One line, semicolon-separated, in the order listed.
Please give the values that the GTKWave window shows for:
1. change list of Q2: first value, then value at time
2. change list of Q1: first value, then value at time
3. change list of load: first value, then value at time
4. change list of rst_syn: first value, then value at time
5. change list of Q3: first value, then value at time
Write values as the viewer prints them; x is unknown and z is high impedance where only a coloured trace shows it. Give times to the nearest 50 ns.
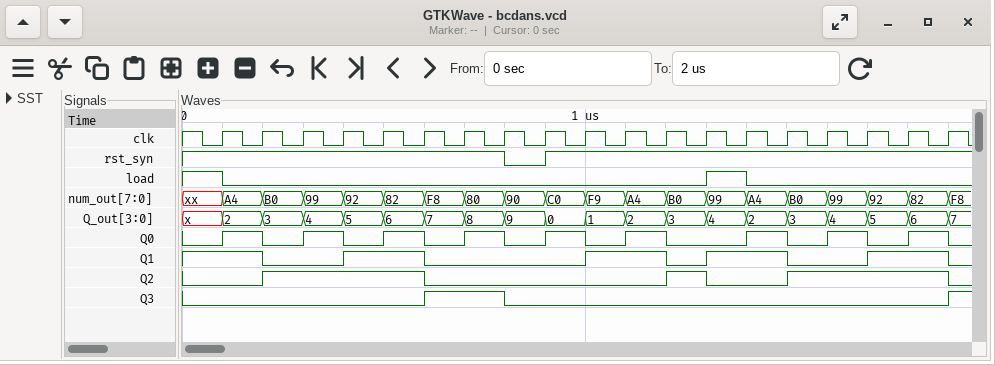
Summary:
0, 1 at 200 ns, 0 at 600 ns, 1 at 1200 ns, 0 at 1300 ns, 1 at 1500 ns, 0 at 1900 ns; 1, 0 at 200 ns, 1 at 400 ns, 0 at 600 ns, 1 at 1000 ns, 0 at 1200 ns, 1 at 1300 ns, 0 at 1500 ns, 1 at 1700 ns, 0 at 1900 ns; 1, 0 at 100 ns, 1 at 1300 ns, 0 at 1400 ns; 1, 0 at 800 ns, 1 at 900 ns; 0, 1 at 600 ns, 0 at 800 ns, 1 at 1900 ns
